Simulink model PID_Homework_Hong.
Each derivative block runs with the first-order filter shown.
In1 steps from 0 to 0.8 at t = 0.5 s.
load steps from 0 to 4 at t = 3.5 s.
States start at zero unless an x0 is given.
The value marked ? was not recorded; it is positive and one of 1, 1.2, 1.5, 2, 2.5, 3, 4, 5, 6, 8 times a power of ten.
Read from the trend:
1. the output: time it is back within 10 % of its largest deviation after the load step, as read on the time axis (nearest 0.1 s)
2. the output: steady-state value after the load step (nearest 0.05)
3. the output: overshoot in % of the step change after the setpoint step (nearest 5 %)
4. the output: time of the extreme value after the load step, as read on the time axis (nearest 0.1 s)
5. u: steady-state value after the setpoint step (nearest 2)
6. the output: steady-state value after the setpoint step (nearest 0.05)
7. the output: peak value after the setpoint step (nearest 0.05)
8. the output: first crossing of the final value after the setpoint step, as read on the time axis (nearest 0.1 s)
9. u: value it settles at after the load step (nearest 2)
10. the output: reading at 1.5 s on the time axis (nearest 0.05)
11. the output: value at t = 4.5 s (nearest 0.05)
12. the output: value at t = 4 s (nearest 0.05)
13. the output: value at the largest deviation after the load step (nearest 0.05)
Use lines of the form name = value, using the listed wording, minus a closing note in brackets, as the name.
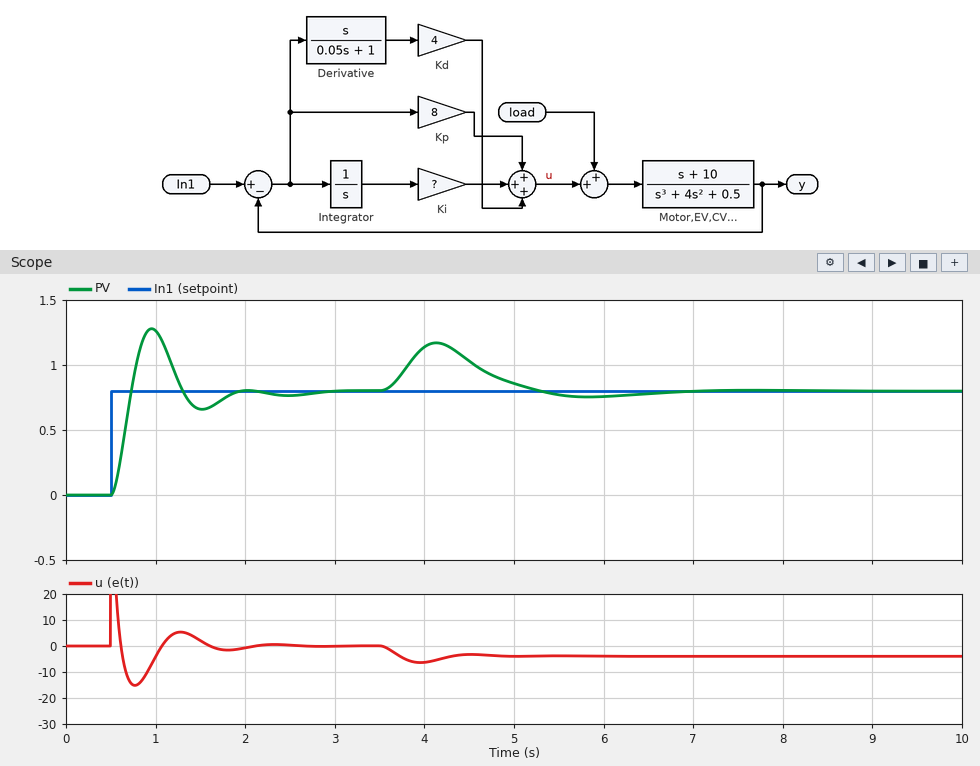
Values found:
the output: time it is back within 10 % of its largest deviation after the load step, as read on the time axis = 6.2 s
the output: steady-state value after the load step = 0.80
the output: overshoot in % of the step change after the setpoint step = 60 %
the output: time of the extreme value after the load step, as read on the time axis = 4.1 s
u: steady-state value after the setpoint step = 0
the output: steady-state value after the setpoint step = 0.80
the output: peak value after the setpoint step = 1.30
the output: first crossing of the final value after the setpoint step, as read on the time axis = 0.7 s
u: value it settles at after the load step = -4
the output: reading at 1.5 s on the time axis = 0.65
the output: value at t = 4.5 s = 1.05
the output: value at t = 4 s = 1.15
the output: value at the largest deviation after the load step = 1.15
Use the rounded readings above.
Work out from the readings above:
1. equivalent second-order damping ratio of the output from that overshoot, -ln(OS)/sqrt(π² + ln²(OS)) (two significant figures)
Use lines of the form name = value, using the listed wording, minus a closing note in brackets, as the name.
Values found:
equivalent second-order damping ratio of the output from that overshoot, -ln(OS)/sqrt(π² + ln²(OS)) = 0.16
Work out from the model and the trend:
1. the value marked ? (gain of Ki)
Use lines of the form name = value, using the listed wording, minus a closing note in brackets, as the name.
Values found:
the value marked ? = 15
